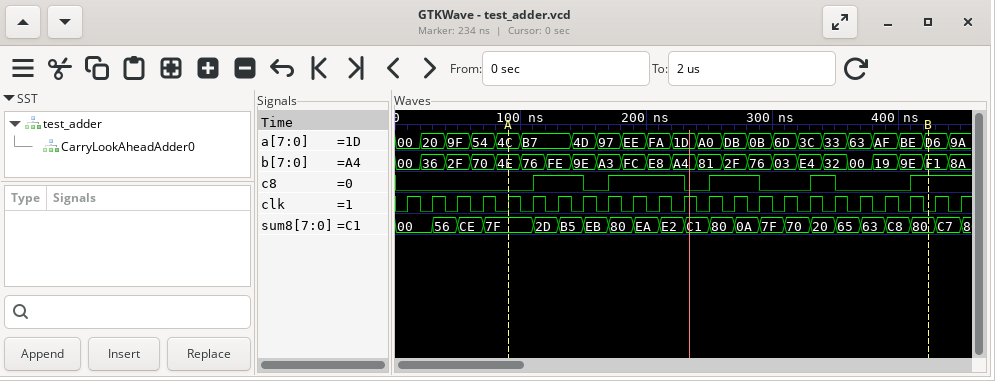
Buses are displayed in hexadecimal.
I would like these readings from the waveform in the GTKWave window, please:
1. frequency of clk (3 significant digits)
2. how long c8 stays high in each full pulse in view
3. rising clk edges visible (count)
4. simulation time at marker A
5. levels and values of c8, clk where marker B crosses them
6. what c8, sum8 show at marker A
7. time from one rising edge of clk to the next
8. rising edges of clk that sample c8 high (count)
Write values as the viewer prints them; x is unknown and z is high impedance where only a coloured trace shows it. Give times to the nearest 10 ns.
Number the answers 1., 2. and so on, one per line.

1. 50.0 MHz
2. 40 ns, 60 ns, 40 ns, 20 ns
3. 23
4. 90 ns
5. c8=1, clk=0
6. c8=0, sum8=7F
7. 20 ns
8. 10
